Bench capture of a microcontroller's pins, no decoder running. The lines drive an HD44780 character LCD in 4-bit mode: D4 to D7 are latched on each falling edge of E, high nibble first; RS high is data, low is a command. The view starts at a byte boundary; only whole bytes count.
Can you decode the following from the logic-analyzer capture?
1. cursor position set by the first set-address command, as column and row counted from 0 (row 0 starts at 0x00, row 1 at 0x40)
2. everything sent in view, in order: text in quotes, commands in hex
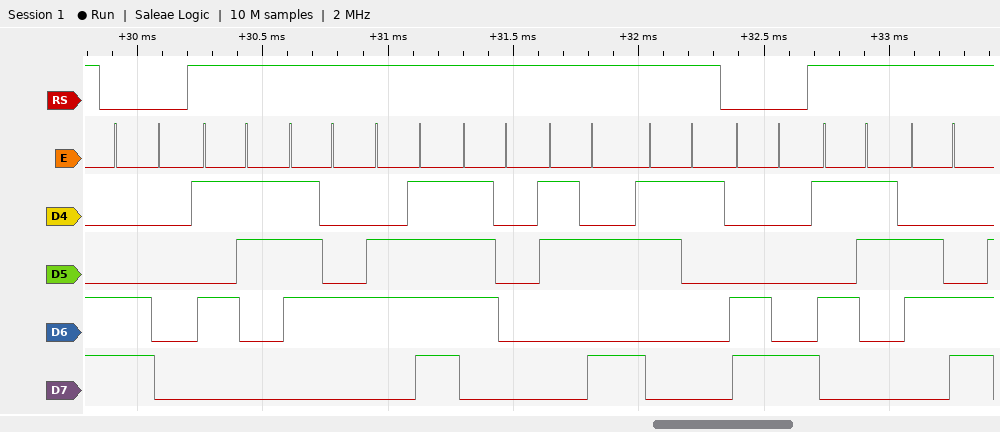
column 0, row 1
0xC0 "Stop:1" 0xC8 "Sl"
